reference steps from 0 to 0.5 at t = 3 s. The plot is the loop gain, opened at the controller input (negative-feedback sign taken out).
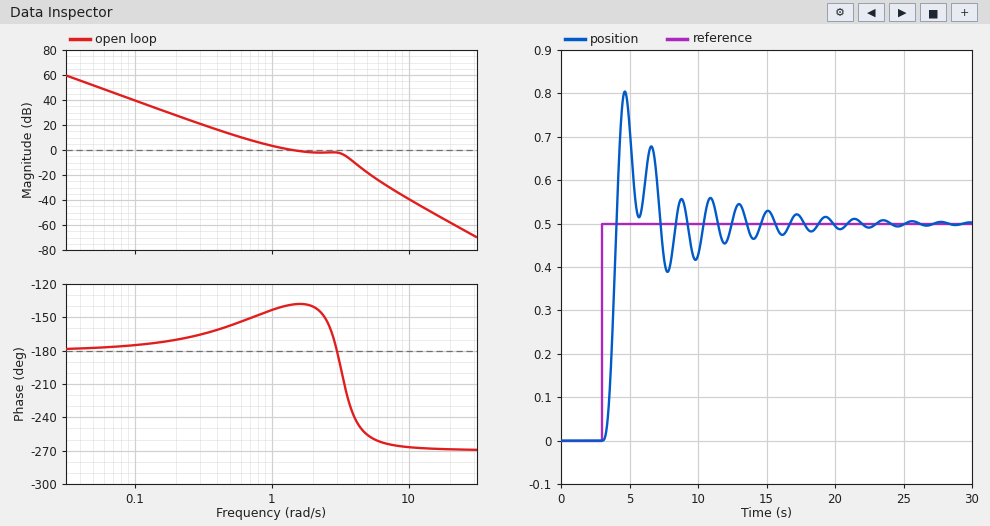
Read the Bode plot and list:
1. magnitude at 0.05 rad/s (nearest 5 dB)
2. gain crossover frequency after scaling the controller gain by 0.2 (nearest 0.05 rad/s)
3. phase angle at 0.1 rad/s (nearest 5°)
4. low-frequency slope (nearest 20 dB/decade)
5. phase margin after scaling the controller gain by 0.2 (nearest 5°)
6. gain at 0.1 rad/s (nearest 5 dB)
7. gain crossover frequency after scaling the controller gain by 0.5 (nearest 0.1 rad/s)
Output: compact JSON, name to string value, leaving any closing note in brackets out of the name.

{"magnitude at 0.05 rad/s": "50 dB", "gain crossover frequency after scaling the controller gain by 0.2": "0.45 rad/s", "phase angle at 0.1 rad/s": "-175°", "low-frequency slope": "-40 dB/decade", "phase margin after scaling the controller gain by 0.2": "20°", "gain at 0.1 rad/s": "40 dB", "gain crossover frequency after scaling the controller gain by 0.5": "0.8 rad/s"}
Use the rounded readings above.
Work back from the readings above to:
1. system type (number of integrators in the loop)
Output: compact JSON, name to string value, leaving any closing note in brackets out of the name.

{"system type": "2"}
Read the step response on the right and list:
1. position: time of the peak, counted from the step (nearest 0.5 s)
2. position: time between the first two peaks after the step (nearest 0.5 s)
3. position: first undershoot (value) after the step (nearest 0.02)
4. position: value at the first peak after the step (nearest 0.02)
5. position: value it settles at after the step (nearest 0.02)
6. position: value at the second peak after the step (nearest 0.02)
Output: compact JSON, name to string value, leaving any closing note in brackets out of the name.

{"position: time of the peak, counted from the step": "1.5 s", "position: time between the first two peaks after the step": "2.0 s", "position: first undershoot (value) after the step": "0.52", "position: value at the first peak after the step": "0.80", "position: value it settles at after the step": "0.50", "position: value at the second peak after the step": "0.68"}
